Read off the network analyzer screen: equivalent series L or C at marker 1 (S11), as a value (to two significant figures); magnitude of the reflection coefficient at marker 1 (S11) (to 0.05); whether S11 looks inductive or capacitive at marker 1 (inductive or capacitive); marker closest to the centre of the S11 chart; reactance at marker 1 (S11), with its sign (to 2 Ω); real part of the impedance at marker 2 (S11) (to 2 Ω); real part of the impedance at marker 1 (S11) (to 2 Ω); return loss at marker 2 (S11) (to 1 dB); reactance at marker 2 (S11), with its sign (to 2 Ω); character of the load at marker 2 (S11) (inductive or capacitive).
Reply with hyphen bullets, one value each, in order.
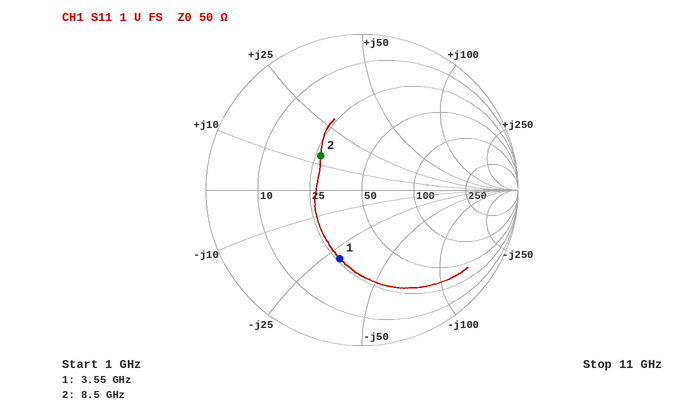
- 1.5 pF
- 0.45
- capacitive
- marker 2
- -30 Ω
- 26 Ω
- 26 Ω
- 9 dB
- +14 Ω
- inductive
